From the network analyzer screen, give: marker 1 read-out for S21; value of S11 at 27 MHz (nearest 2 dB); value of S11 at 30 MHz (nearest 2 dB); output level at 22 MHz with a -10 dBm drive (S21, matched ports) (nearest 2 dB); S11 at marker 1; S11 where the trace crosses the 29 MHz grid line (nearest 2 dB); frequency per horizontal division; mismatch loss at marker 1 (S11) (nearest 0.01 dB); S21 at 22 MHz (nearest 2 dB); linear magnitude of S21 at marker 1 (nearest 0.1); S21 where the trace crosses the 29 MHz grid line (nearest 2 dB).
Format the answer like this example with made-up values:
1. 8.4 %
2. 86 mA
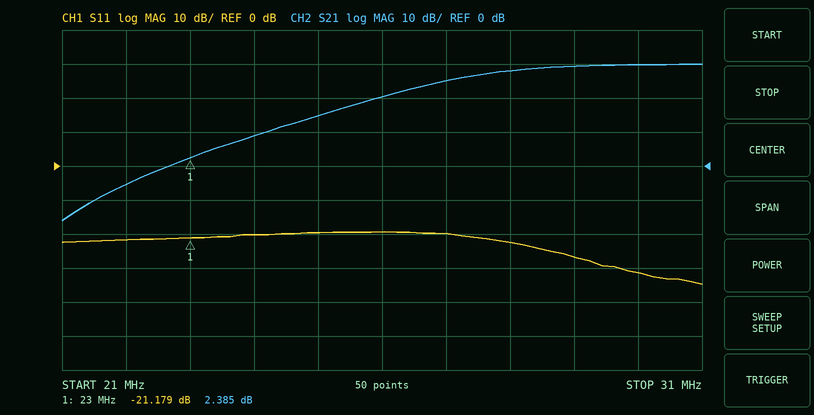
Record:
1. 2.385 dB
2. -20 dB
3. -32 dB
4. -16 dBm
5. -21.179 dB
6. -26 dB
7. 1 MHz
8. 0.03 dB
9. -6 dB
10. 1.3
11. 30 dB
